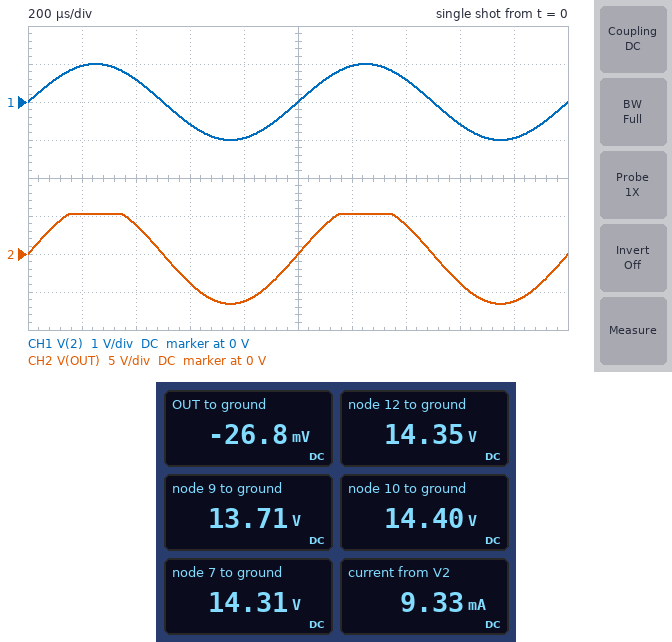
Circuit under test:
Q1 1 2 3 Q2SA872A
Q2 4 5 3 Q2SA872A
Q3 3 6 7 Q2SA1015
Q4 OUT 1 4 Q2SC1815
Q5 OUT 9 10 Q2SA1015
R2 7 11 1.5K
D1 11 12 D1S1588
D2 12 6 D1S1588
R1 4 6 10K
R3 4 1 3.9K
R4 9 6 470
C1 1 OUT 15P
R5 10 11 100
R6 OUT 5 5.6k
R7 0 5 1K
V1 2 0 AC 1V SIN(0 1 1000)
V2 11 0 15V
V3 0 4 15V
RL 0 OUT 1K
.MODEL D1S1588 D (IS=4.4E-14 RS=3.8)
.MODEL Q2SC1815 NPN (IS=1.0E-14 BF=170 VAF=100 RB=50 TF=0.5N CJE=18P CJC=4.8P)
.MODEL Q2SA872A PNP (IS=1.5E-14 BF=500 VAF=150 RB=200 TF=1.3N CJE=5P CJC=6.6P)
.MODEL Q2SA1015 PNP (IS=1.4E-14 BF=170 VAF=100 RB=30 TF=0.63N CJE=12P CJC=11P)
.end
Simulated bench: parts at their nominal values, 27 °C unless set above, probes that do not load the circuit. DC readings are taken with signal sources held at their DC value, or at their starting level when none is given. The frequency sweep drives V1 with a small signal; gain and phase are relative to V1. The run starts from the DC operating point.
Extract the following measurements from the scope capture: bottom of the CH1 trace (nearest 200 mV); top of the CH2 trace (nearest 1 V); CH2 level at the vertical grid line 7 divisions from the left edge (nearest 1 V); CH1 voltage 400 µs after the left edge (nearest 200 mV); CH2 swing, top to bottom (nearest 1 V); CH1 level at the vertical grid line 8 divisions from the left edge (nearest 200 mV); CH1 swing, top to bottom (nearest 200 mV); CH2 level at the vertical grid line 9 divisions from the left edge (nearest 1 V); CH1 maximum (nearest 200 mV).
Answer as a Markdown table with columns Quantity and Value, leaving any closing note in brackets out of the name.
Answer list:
| Quantity | Value |
|---|---|
| bottom of the CH1 trace | -1.0 V |
| top of the CH2 trace | 5 V |
| CH2 level at the vertical grid line 7 divisions from the left edge | 4 V |
| CH1 voltage 400 µs after the left edge | 600 mV |
| CH2 swing, top to bottom | 12 V |
| CH1 level at the vertical grid line 8 divisions from the left edge | -600 mV |
| CH1 swing, top to bottom | 2.0 V |
| CH2 level at the vertical grid line 9 divisions from the left edge | -6 V |
| CH1 maximum | 1.0 V |
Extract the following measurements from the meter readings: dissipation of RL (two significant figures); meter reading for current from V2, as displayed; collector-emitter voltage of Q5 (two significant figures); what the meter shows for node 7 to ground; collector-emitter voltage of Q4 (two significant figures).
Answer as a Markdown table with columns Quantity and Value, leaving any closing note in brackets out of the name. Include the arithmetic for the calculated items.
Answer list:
| Quantity | Value |
|---|---|
| dissipation of RL | (0 V - (-26.8 mV))^2 / 1 kΩ = 720 nW |
| meter reading for current from V2, as displayed | 9.33 mA |
| collector-emitter voltage of Q5 | -26.8 mV - 14.4 V = -14 V |
| what the meter shows for node 7 to ground | 14.31 V |
| collector-emitter voltage of Q4 | -26.8 mV - (-15 V) = 15 V |
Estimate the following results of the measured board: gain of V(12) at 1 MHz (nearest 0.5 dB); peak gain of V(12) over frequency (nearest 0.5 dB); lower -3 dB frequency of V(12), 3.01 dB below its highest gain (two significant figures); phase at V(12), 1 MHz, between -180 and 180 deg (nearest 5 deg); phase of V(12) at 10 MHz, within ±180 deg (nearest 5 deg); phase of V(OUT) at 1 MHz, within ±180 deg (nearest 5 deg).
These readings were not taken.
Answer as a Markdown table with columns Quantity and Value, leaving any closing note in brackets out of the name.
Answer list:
| Quantity | Value |
|---|---|
| gain of V(12) at 1 MHz | -52.0 dB |
| peak gain of V(12) over frequency | -33.0 dB |
| lower -3 dB frequency of V(12), 3.01 dB below its highest gain | 82 MHz |
| phase at V(12), 1 MHz, between -180 and 180 deg | 80 deg |
| phase of V(12) at 10 MHz, within ±180 deg | -30 deg |
| phase of V(OUT) at 1 MHz, within ±180 deg | -10 deg |
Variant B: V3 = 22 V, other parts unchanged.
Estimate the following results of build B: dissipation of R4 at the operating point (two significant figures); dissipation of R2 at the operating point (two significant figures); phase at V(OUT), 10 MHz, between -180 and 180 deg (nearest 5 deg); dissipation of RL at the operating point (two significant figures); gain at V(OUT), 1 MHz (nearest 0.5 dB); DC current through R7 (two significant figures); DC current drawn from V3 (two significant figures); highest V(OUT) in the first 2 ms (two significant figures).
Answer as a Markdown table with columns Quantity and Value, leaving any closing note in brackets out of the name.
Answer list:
| Quantity | Value |
|---|---|
| dissipation of R4 at the operating point | 480 nW |
| dissipation of R2 at the operating point | 330 µW |
| phase at V(OUT), 10 MHz, between -180 and 180 deg | -105 deg |
| dissipation of RL at the operating point | 1.3 µW |
| gain at V(OUT), 1 MHz | 16.5 dB |
| DC current through R7 | 5.1 µA |
| DC current drawn from V3 | 10 mA |
| highest V(OUT) in the first 2 ms | 5.3 V |
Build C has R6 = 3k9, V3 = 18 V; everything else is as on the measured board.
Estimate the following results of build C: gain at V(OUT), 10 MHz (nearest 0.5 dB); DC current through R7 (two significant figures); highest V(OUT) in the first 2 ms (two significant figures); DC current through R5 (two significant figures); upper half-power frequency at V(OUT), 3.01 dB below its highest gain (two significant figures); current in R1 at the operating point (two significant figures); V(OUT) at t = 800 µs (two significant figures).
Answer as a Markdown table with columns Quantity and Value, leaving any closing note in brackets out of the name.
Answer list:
| Quantity | Value |
|---|---|
| gain at V(OUT), 10 MHz | 12.5 dB |
| DC current through R7 | 4.3 µA |
| highest V(OUT) in the first 2 ms | 4.8 V |
| DC current through R5 | 6.1 mA |
| upper half-power frequency at V(OUT), 3.01 dB below its highest gain | 11 MHz |
| current in R1 at the operating point | 3.2 mA |
| V(OUT) at t = 800 µs | -4.6 V |
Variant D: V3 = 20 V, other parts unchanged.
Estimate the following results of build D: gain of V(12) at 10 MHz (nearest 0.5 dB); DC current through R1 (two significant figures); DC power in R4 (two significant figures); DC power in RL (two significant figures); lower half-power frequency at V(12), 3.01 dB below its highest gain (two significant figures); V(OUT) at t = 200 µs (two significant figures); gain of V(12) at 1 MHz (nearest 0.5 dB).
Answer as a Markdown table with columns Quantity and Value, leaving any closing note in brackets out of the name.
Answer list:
| Quantity | Value |
|---|---|
| gain of V(12) at 10 MHz | -39.5 dB |
| DC current through R1 | 3.4 mA |
| DC power in R4 | 470 nW |
| DC power in RL | 1.1 µW |
| lower half-power frequency at V(12), 3.01 dB below its highest gain | 85 MHz |
| V(OUT) at t = 200 µs | 5.3 V |
| gain of V(12) at 1 MHz | -53.0 dB |
